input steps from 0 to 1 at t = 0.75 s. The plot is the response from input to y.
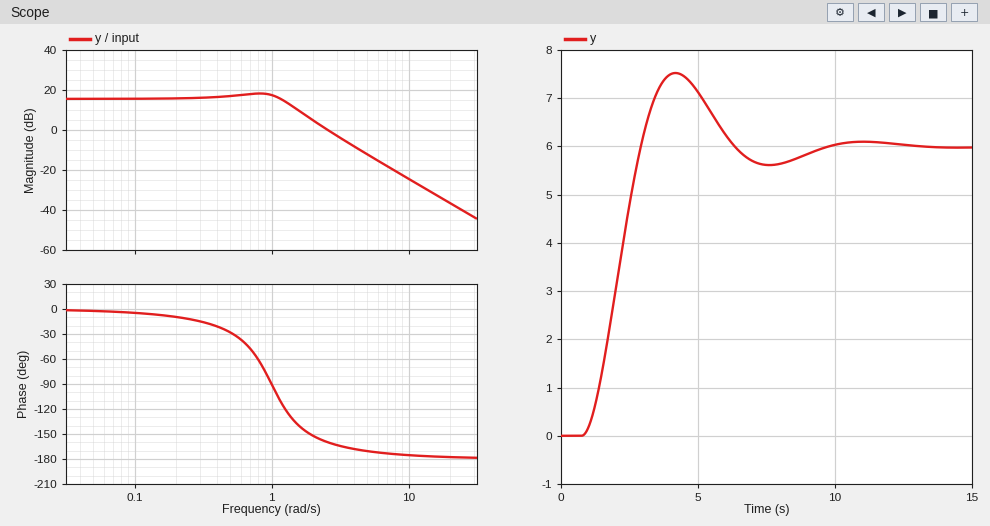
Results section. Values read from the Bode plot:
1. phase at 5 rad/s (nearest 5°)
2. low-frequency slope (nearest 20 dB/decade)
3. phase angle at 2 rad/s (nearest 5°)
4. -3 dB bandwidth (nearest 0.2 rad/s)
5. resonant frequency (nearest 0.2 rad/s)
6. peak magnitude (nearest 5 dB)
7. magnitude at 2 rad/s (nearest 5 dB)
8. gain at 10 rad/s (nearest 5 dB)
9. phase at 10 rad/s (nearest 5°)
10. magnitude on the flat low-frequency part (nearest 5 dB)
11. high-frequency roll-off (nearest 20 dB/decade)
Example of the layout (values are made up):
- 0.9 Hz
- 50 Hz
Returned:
- -170°
- 0 dB/decade
- -150°
- 1.4 rad/s
- 0.8 rad/s
- 20 dB
- 5 dB
- -25 dB
- -175°
- 15 dB
- -40 dB/decade
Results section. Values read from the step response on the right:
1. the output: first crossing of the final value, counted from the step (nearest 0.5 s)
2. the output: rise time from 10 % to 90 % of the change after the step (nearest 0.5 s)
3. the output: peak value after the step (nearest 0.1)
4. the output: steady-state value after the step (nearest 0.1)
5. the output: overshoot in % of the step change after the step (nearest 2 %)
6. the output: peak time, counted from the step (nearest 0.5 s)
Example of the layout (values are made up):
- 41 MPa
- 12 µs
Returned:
- 2.0 s
- 1.5 s
- 7.5
- 6.0
- 26 %
- 3.5 s
